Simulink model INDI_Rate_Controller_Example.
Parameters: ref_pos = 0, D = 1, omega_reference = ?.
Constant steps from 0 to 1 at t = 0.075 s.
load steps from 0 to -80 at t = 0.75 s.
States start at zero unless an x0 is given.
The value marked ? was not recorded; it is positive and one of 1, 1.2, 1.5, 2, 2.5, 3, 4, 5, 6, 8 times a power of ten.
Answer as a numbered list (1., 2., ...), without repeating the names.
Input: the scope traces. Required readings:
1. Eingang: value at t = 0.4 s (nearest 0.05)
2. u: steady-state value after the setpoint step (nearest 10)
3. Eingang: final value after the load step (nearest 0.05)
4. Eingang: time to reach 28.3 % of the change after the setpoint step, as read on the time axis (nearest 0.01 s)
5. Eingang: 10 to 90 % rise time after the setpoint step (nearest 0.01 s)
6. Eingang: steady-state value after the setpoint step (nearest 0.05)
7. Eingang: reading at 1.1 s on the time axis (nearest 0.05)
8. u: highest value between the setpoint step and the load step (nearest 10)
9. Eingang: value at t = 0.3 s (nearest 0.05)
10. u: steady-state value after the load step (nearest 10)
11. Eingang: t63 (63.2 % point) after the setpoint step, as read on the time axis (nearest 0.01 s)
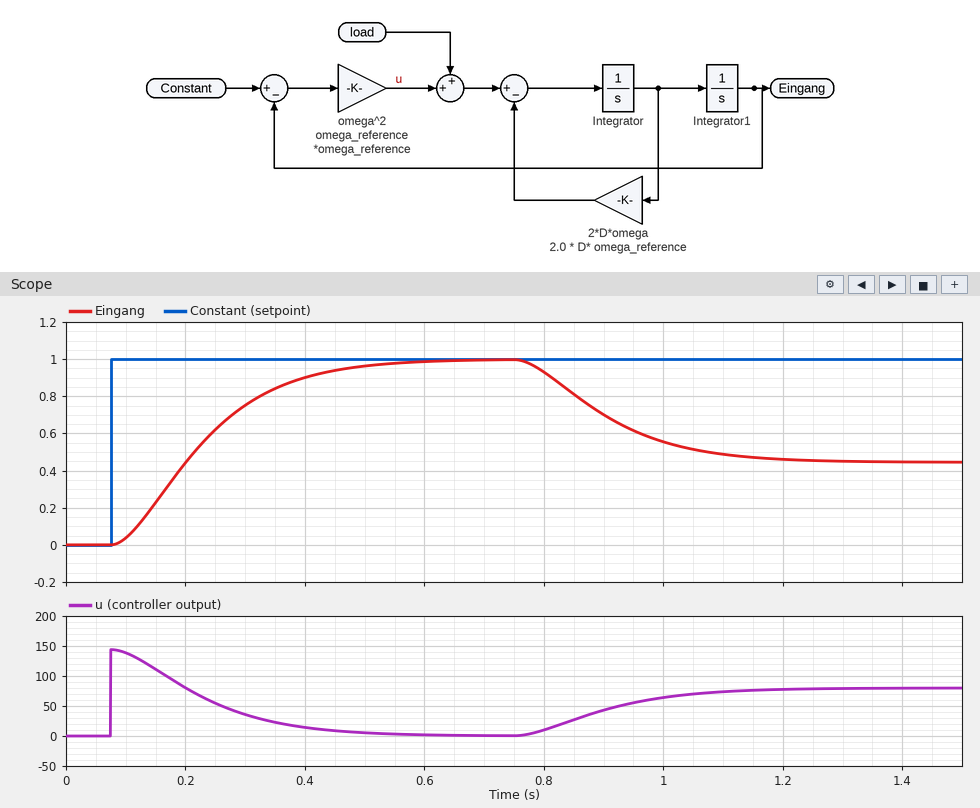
1. 0.90
2. 0
3. 0.45
4. 0.16 s
5. 0.28 s
6. 1.00
7. 0.50
8. 140
9. 0.75
10. 80
11. 0.25 s
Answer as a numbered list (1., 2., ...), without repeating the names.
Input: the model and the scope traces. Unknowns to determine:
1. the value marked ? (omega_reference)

1. 12
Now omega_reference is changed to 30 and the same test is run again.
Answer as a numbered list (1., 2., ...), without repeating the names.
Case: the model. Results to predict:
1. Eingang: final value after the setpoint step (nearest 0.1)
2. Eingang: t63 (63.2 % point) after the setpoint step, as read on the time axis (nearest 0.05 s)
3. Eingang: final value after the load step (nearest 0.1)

1. 1.0
2. 0.15 s
3. 0.9
